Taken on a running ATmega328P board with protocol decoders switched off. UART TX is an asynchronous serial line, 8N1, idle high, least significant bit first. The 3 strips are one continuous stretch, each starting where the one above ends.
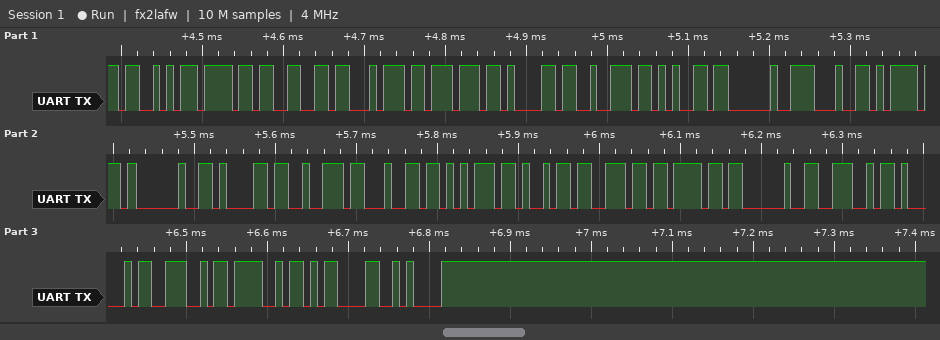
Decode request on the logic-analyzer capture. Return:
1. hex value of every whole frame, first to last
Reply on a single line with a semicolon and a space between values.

53 6F 66 74 77 61 72 65 20 64 6F 20 61 72 64 75 69 6E 6F 20 4E 41 4E 4F 0D 0A
